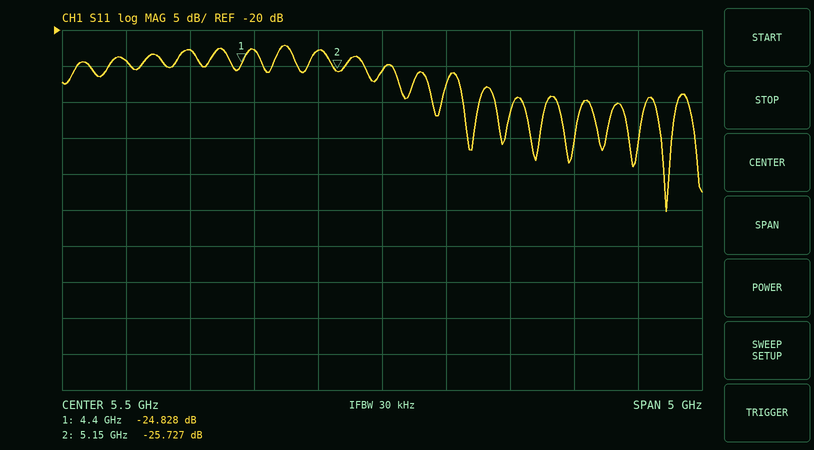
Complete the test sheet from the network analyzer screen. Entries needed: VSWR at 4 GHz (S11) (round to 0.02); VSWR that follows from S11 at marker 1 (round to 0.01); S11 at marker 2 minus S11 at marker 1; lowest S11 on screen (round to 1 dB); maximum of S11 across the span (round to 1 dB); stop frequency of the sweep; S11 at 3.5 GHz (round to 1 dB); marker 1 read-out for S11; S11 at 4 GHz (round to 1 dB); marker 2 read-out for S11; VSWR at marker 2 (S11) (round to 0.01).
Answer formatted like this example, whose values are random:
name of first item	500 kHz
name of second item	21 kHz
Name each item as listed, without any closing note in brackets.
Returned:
VSWR at 4 GHz (S11)	1.16
VSWR that follows from S11 at marker 1	1.12
S11 at marker 2 minus S11 at marker 1	-0.899 dB
lowest S11 on screen	-45 dB
maximum of S11 across the span	-22 dB
stop frequency of the sweep	8 GHz
S11 at 3.5 GHz	-24 dB
marker 1 read-out for S11	-24.828 dB
S11 at 4 GHz	-23 dB
marker 2 read-out for S11	-25.727 dB
VSWR at marker 2 (S11)	1.11
